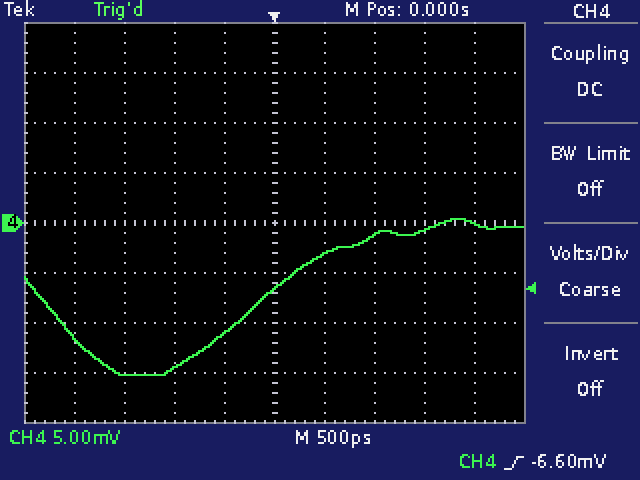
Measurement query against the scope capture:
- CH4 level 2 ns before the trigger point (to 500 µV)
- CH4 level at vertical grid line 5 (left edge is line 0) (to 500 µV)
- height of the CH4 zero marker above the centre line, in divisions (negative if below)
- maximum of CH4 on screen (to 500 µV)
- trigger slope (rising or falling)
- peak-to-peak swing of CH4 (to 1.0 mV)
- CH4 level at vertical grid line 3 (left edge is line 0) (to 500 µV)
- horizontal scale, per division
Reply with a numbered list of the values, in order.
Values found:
1. -11.5 mV
2. -6.5 mV
3. 0.0 div
4. 500 µV
5. rising
6. 16.0 mV
7. -14.5 mV
8. 500 ps
